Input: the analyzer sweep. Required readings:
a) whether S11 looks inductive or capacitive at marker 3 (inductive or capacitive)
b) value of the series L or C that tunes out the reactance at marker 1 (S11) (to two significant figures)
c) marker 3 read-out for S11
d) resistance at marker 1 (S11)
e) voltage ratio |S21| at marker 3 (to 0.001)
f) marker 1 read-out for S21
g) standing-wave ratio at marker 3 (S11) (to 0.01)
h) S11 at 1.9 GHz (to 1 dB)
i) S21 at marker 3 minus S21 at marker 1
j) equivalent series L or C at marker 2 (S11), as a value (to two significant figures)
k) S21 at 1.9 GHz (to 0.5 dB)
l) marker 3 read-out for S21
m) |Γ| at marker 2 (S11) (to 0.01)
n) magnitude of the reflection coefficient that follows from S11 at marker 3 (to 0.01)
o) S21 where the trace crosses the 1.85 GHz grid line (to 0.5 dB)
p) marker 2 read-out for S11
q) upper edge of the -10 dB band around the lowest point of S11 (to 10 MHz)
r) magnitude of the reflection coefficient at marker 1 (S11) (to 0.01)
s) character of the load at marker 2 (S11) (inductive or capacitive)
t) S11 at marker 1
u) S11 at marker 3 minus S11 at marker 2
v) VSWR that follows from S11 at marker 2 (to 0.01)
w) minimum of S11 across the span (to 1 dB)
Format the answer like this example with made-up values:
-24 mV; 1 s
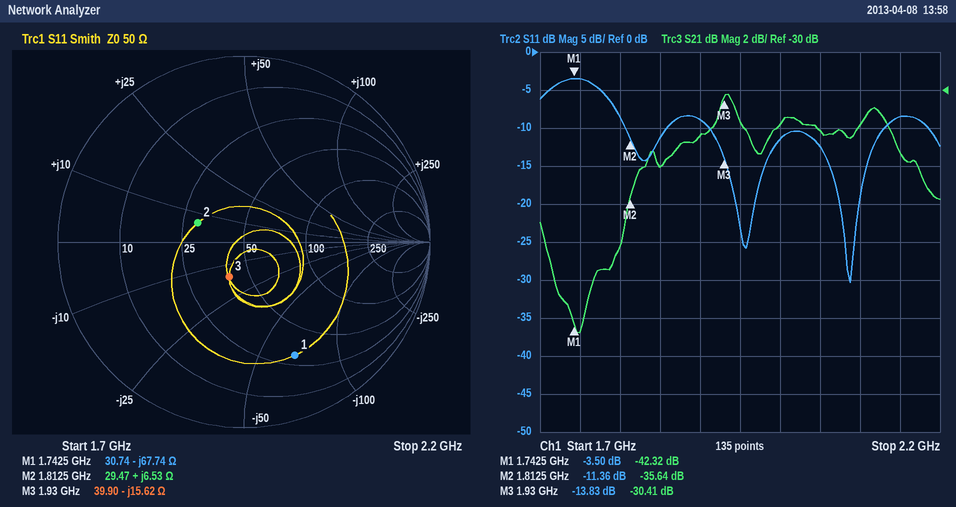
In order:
capacitive; 6.2 nH; -13.83 dB; 30.74 Ω; 0.030; -42.32 dB; 1.51; -9 dB; 11.91 dB; 570 pH; -32.5 dB; -30.41 dB; 0.27; 0.20; -34.0 dB; -11.36 dB; 2.13 GHz; 0.67; inductive; -3.50 dB; -2.47 dB; 1.74; -30 dB
